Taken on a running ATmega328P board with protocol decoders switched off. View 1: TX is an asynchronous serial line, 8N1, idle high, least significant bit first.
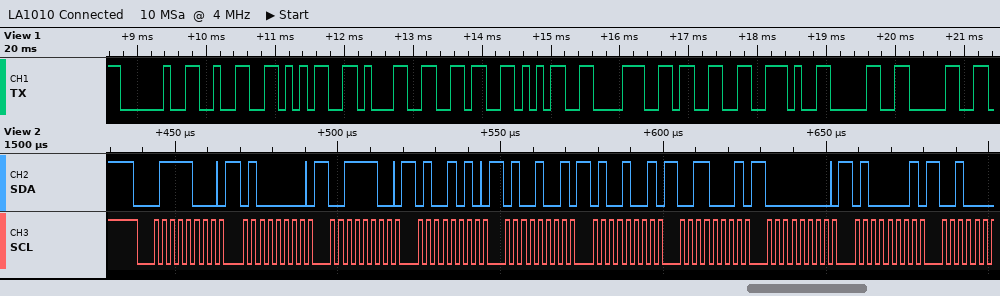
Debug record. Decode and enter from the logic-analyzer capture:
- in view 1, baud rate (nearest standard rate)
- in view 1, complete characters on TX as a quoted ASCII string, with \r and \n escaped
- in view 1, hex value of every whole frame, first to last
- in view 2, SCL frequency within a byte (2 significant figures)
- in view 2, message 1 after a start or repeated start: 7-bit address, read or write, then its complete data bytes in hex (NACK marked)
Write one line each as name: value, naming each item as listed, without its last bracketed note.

in view 1, baud rate: 9600 baud
in view 1, complete characters on TX as a quoted ASCII string, with \r and \n escaped: " 2516583.00"
in view 1, hex value of every whole frame, first to last: 20 32 35 31 36 35 38 33 2E 30 30
in view 2, SCL frequency within a byte: 400 kHz
in view 2, message 1 after a start or repeated start: 7-bit address, read or write, then its complete data bytes in hex: 0x3C write: 40 3C 4A 49 49 31 00 41
